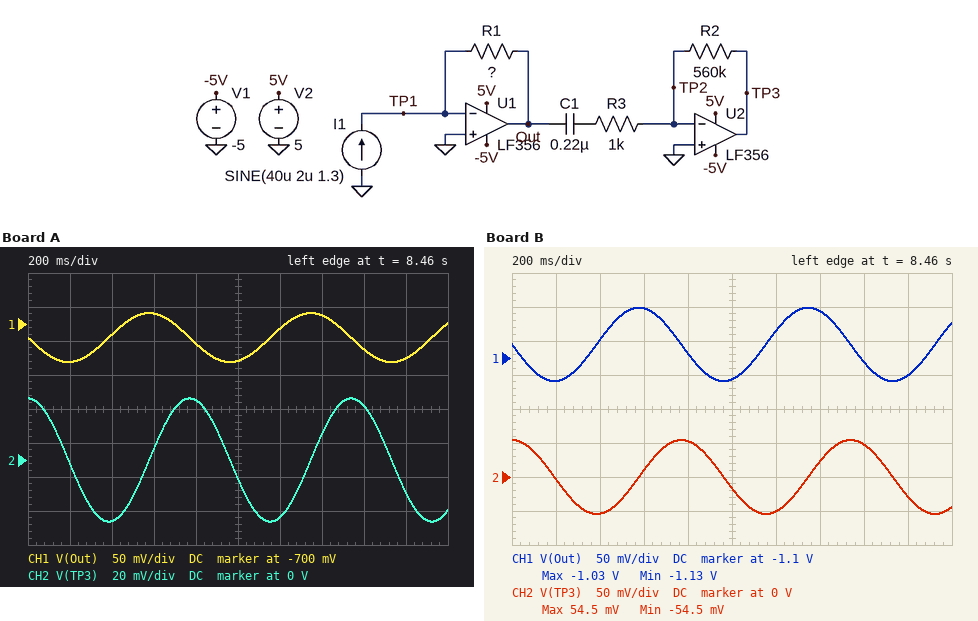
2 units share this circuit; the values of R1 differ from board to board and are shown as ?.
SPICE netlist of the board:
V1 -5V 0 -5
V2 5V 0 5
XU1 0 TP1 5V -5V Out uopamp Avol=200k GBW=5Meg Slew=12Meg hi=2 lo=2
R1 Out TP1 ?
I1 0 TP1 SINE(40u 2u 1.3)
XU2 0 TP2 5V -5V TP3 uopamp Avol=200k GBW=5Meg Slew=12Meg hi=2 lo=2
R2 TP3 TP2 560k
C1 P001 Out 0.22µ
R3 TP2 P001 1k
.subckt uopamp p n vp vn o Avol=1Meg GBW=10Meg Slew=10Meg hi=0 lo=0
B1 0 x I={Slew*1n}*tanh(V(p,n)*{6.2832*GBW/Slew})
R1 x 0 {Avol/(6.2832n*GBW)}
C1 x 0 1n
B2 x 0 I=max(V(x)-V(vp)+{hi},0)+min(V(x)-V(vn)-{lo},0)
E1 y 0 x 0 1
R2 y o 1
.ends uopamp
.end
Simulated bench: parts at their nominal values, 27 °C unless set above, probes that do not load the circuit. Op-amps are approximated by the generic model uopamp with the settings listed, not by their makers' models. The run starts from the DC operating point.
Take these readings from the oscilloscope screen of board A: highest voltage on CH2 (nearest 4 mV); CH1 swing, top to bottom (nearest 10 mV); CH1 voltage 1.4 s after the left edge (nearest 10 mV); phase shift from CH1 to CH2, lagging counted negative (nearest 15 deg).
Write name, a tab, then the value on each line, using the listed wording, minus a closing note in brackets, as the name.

highest voltage on CH2	36 mV
CH1 swing, top to bottom	70 mV
CH1 voltage 1.4 s after the left edge	-690 mV
phase shift from CH1 to CH2, lagging counted negative	-90 deg
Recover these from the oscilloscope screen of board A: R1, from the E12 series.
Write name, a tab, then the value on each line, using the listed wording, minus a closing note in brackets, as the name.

R1, from the E12 series	18 kΩ
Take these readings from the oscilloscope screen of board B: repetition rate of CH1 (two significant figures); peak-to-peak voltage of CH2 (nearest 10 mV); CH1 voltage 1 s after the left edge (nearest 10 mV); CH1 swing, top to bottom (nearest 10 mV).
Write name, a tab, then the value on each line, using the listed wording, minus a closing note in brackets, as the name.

repetition rate of CH1	1.3 Hz
peak-to-peak voltage of CH2	110 mV
CH1 voltage 1 s after the left edge	-1.13 V
CH1 swing, top to bottom	110 mV
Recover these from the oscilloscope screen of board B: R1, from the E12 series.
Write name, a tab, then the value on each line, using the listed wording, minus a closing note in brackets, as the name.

R1, from the E12 series	27 kΩ
